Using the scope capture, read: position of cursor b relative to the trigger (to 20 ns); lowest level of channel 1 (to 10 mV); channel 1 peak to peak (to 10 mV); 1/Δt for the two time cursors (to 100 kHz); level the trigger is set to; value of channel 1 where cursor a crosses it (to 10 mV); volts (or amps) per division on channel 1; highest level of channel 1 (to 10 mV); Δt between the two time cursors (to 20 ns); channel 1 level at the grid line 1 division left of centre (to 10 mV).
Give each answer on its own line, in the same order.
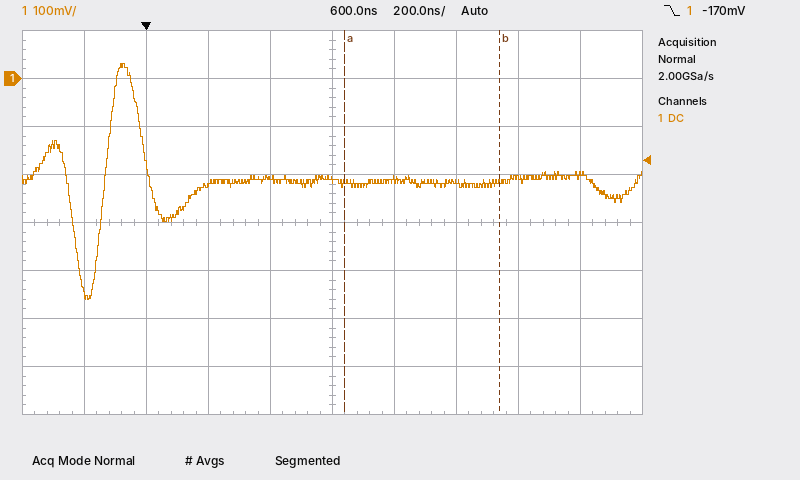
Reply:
+1.14 µs
-460 mV
490 mV
2.0 MHz
-170 mV
-220 mV
100 mV
30 mV
500 ns
-210 mV
